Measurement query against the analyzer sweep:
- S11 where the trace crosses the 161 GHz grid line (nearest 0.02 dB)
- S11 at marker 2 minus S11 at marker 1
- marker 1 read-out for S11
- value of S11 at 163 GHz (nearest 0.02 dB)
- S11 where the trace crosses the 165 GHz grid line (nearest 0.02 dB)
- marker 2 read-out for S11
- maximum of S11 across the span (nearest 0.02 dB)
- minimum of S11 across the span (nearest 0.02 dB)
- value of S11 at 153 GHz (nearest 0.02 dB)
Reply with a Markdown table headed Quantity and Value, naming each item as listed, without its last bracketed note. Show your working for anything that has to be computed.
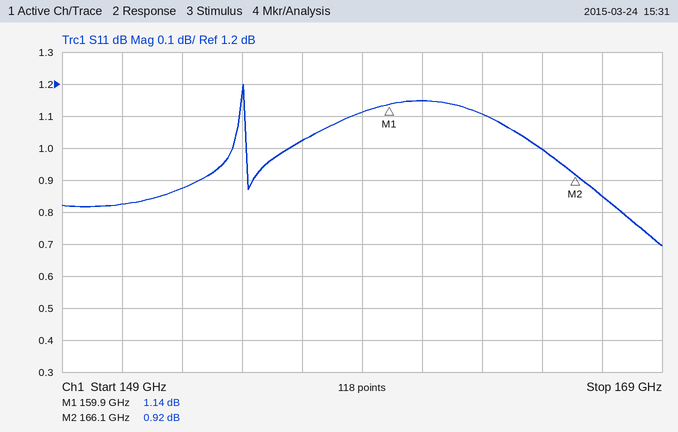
| Quantity | Value |
|---|---|
| S11 where the trace crosses the 161 GHz grid line | 1.14 dB |
| S11 at marker 2 minus S11 at marker 1 | 0.92 − (1.14) = -0.22 dB |
| marker 1 read-out for S11 | 1.14 dB |
| value of S11 at 163 GHz | 1.10 dB |
| S11 where the trace crosses the 165 GHz grid line | 1.00 dB |
| marker 2 read-out for S11 | 0.92 dB |
| maximum of S11 across the span | 1.20 dB |
| minimum of S11 across the span | 0.70 dB |
| value of S11 at 153 GHz | 0.88 dB |
